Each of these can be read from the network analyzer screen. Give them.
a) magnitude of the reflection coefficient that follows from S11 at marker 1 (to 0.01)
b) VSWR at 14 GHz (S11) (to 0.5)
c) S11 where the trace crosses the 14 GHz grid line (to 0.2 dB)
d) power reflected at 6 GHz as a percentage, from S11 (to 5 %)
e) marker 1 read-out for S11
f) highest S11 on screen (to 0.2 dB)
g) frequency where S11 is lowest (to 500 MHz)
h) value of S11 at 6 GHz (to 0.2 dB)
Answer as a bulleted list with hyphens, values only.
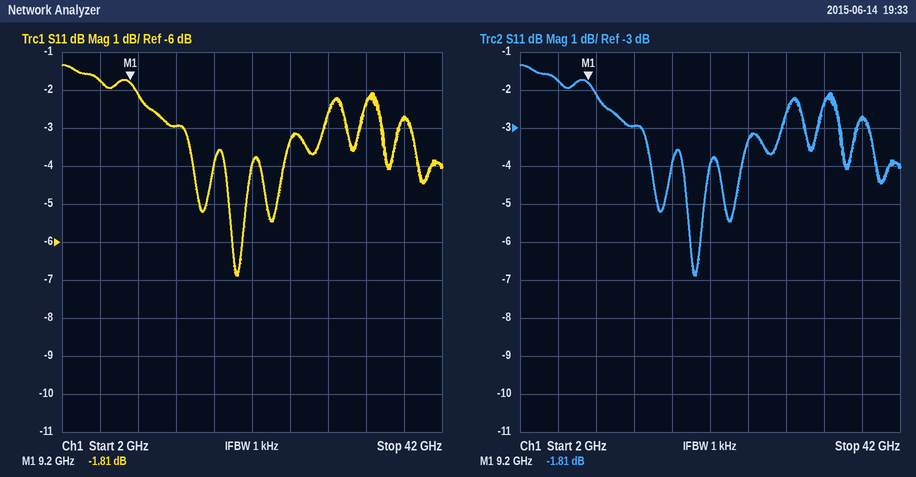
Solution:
- 0.81
- 6.0
- -3.0 dB
- 65 %
- -1.81 dB
- -1.4 dB
- 20.5 GHz
- -1.8 dB
